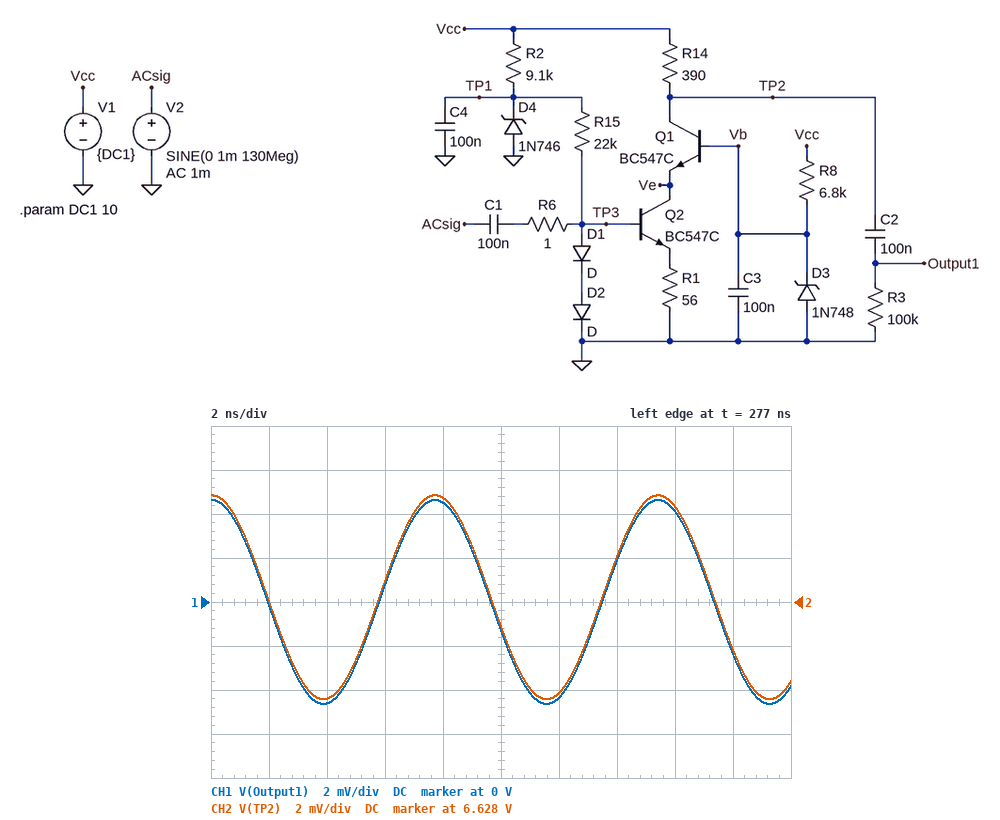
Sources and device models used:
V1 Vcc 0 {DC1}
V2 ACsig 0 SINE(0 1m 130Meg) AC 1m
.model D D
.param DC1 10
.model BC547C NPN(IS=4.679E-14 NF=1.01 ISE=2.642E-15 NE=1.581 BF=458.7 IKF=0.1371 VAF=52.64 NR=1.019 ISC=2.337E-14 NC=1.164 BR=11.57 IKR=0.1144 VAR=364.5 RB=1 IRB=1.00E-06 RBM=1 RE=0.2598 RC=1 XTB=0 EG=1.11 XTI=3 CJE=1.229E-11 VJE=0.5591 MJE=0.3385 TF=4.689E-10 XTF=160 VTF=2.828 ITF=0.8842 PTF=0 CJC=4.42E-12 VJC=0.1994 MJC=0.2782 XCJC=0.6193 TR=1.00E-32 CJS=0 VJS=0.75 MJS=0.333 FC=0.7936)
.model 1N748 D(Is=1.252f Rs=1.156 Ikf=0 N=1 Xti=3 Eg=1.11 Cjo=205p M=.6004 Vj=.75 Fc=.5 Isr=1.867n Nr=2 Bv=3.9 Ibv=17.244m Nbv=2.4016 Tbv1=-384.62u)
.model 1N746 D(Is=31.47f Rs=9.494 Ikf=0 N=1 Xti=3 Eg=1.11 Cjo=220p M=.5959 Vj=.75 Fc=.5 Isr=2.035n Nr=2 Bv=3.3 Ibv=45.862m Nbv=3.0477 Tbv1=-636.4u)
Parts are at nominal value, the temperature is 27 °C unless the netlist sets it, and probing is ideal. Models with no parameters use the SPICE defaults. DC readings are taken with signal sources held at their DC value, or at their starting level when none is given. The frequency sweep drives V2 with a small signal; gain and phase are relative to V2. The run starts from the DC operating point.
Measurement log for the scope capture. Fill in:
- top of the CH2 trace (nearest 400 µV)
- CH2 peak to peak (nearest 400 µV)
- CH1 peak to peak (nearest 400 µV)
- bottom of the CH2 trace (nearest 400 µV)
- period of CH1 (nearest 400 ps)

6.6328 V
9.2 mV
9.2 mV
6.6236 V
7.6 ns
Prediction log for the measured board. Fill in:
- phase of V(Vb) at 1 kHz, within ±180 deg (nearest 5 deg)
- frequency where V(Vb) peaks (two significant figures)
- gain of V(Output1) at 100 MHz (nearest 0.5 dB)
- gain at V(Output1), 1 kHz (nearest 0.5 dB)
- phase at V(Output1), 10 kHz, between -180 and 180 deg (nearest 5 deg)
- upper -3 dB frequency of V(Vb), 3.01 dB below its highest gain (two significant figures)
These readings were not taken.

-120 deg
6.9 kHz
14.5 dB
9.0 dB
-170 deg
27 kHz
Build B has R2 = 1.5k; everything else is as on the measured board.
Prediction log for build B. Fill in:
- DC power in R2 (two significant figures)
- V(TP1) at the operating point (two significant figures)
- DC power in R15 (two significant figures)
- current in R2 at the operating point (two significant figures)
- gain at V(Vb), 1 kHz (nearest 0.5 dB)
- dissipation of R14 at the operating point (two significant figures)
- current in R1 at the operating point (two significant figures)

31 mW
3.2 V
180 µW
4.6 mA
-59.0 dB
30 mW
8.8 mA
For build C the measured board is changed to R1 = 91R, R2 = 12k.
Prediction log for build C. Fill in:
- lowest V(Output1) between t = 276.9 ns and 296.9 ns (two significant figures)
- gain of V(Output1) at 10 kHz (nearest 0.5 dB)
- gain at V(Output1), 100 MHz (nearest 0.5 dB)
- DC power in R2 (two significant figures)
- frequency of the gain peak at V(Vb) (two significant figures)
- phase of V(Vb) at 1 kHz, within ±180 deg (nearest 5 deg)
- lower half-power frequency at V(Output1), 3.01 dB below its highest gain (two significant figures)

-3.0 mV
12.0 dB
10.5 dB
4.1 mW
7.2 kHz
-115 deg
2.2 kHz
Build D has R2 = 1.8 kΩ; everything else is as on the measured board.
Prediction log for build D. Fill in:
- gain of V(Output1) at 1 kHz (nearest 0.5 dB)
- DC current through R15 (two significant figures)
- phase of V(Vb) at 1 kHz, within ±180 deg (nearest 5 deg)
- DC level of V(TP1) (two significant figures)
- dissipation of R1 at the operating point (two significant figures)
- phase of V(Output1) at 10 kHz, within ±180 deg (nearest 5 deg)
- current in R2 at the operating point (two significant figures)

8.5 dB
89 µA
-115 deg
3.1 V
4.3 mW
-165 deg
3.8 mA
